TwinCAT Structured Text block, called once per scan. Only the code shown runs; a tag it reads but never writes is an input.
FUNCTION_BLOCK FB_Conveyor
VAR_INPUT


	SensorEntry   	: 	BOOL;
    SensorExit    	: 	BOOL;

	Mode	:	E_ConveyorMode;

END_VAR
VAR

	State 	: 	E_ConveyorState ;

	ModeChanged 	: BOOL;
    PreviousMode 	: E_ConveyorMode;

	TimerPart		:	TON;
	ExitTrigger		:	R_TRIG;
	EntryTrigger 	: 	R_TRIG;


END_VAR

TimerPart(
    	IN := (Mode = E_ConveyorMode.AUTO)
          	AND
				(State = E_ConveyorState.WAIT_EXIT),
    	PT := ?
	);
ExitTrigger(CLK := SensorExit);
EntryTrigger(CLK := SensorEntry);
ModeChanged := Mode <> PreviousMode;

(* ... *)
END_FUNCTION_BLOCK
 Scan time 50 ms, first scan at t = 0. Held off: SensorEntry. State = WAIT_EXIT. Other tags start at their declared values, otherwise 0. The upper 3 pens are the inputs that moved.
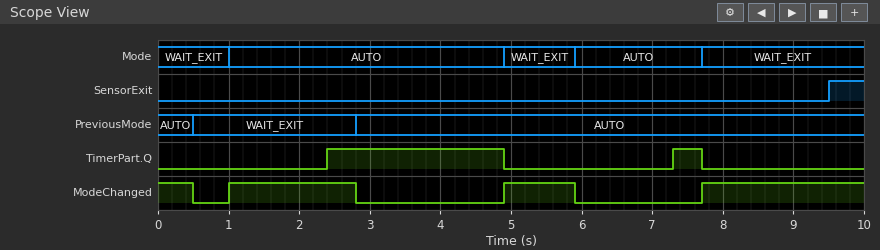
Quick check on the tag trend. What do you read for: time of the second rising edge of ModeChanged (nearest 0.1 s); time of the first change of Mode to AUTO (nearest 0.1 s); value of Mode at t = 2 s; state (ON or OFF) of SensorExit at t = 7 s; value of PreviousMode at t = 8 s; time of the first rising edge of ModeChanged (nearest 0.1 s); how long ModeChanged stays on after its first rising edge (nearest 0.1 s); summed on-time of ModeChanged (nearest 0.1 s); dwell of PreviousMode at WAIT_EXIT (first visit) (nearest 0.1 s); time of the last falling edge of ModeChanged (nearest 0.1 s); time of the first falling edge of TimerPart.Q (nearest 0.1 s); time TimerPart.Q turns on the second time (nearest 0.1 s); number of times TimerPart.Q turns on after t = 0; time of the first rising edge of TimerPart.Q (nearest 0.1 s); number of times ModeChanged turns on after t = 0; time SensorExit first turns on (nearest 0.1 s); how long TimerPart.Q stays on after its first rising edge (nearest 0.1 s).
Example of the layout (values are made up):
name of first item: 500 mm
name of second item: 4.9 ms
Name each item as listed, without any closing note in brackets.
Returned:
time of the second rising edge of ModeChanged: 4.9 s
time of the first change of Mode to AUTO: 1.0 s
value of Mode at t = 2 s: AUTO
state (ON or OFF) of SensorExit at t = 7 s: OFF
value of PreviousMode at t = 8 s: AUTO
time of the first rising edge of ModeChanged: 1.0 s
how long ModeChanged stays on after its first rising edge: 1.8 s
summed on-time of ModeChanged: 5.6 s
dwell of PreviousMode at WAIT_EXIT (first visit): 2.3 s
time of the last falling edge of ModeChanged: 5.9 s
time of the first falling edge of TimerPart.Q: 4.9 s
time TimerPart.Q turns on the second time: 7.3 s
number of times TimerPart.Q turns on after t = 0: 2
time of the first rising edge of TimerPart.Q: 2.4 s
number of times ModeChanged turns on after t = 0: 3
time SensorExit first turns on: 9.5 s
how long TimerPart.Q stays on after its first rising edge: 2.5 s
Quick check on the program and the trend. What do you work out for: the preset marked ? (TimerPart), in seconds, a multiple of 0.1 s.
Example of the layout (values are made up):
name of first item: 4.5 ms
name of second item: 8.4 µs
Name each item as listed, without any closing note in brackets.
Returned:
the preset marked ? (TimerPart), in seconds, a multiple of 0.1 s: 1.4 s
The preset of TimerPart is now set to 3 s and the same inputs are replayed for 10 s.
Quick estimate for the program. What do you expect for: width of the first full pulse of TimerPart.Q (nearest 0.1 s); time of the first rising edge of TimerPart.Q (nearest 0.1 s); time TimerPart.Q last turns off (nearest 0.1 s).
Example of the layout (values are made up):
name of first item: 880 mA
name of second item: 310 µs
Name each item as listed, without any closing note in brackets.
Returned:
width of the first full pulse of TimerPart.Q: 0.9 s
time of the first rising edge of TimerPart.Q: 4.0 s
time TimerPart.Q last turns off: 4.9 s
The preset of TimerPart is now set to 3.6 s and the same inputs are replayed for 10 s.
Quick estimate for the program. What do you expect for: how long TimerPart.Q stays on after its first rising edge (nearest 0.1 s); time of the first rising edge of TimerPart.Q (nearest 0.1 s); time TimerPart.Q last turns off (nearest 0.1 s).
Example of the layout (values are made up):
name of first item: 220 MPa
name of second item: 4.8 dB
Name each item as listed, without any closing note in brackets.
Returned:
how long TimerPart.Q stays on after its first rising edge: 0.3 s
time of the first rising edge of TimerPart.Q: 4.6 s
time TimerPart.Q last turns off: 4.9 s
